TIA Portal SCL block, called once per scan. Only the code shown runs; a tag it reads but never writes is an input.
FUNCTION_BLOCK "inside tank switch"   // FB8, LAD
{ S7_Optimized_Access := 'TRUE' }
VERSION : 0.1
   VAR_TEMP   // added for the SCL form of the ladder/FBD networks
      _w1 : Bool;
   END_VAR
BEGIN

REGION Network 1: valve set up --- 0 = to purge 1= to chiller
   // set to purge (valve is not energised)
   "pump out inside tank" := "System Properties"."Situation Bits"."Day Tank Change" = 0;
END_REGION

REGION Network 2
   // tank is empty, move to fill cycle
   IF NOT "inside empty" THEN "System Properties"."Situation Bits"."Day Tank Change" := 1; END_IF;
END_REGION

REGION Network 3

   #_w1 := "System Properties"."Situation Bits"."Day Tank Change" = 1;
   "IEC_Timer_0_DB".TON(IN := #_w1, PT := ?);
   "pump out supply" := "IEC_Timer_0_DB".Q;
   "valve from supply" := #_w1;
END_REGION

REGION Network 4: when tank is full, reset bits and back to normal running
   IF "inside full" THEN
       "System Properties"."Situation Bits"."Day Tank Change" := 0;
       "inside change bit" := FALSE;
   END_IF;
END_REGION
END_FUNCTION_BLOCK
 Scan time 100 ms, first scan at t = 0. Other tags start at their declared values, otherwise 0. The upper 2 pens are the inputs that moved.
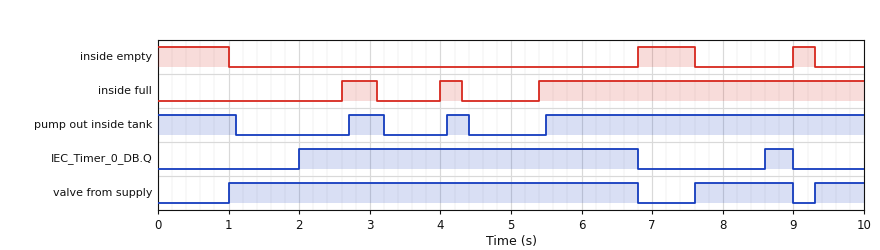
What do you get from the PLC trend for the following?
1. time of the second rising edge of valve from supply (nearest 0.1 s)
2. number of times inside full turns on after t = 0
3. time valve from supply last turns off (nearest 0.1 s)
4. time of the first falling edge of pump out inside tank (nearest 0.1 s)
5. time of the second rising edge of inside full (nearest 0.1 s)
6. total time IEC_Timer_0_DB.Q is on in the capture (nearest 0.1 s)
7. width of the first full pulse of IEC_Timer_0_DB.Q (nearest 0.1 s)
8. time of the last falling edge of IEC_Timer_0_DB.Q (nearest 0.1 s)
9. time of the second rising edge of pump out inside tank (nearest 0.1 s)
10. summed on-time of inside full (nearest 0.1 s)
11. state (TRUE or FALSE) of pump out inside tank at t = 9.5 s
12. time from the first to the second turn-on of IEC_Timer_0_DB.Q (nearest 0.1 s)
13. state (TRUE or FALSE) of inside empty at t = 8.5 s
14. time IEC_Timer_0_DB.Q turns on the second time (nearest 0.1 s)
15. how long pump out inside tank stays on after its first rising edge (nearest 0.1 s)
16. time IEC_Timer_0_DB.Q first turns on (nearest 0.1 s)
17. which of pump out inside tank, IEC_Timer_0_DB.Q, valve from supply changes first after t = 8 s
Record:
7.6 s
3
9.0 s
1.1 s
4.0 s
5.2 s
4.8 s
9.0 s
4.1 s
5.4 s
TRUE
6.6 s
FALSE
8.6 s
0.5 s
2.0 s
IEC_Timer_0_DB.Q
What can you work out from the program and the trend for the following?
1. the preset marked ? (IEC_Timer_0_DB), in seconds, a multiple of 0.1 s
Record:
1.0 s
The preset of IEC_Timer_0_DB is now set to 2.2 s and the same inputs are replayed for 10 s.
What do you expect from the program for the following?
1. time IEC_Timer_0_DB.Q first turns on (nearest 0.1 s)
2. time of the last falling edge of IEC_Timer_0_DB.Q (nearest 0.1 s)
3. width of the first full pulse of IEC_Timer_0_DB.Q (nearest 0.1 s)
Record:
3.2 s
6.8 s
3.6 s
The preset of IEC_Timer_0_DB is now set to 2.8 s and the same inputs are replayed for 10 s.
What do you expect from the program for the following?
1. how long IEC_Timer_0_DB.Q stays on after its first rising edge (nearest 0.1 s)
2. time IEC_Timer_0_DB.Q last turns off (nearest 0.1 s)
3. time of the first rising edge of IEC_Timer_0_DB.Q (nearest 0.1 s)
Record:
3.0 s
6.8 s
3.8 s
